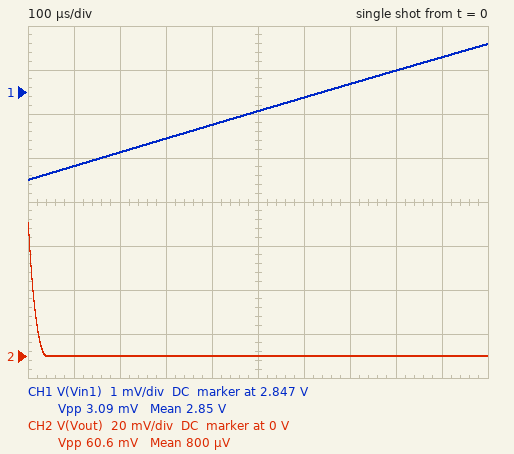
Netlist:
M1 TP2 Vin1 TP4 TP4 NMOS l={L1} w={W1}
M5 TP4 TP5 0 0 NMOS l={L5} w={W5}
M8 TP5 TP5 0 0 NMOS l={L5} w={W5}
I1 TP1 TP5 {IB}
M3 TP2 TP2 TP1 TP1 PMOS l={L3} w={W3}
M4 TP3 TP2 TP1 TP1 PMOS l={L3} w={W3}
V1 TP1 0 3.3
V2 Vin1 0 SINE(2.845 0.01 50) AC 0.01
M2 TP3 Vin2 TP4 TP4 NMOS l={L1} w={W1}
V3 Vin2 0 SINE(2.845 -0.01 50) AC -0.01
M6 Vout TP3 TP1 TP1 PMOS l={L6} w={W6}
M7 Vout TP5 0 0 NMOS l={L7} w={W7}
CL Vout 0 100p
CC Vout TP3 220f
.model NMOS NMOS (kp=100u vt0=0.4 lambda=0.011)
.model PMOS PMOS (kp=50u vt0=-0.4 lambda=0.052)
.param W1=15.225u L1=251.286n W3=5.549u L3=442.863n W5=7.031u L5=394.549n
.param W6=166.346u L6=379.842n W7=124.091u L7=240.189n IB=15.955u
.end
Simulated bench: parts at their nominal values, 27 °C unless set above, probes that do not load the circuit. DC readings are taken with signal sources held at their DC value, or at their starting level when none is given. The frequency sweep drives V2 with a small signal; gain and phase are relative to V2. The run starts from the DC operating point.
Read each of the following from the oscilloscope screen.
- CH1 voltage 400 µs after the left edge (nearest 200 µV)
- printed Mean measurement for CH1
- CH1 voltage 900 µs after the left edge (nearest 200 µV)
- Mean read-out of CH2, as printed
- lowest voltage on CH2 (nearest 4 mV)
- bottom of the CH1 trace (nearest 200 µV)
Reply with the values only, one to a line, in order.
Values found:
2.8462 V
2.85 V
2.8478 V
800 µV
0 V
2.8450 V
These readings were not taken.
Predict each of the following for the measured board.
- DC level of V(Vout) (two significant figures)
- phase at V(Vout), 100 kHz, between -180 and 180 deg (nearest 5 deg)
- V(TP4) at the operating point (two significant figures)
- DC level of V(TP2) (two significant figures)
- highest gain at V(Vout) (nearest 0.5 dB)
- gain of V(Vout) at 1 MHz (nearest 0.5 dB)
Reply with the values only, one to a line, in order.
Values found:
61 mV
150 deg
2.4 V
2.7 V
56.5 dB
41.0 dB
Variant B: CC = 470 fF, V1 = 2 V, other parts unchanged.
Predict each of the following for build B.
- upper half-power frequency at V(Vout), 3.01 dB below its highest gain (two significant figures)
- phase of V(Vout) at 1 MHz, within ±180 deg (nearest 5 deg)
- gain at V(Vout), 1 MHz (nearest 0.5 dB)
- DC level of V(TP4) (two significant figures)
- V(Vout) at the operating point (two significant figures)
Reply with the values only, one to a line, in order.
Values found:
5.8 MHz
170 deg
-58.0 dB
1.4 V
55 mV
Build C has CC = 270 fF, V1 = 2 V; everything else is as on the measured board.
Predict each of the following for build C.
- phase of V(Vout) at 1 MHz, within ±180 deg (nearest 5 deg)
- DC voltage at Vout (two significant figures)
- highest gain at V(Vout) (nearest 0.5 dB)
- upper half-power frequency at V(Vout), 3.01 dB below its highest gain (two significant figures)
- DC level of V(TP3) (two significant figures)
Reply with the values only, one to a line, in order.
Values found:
170 deg
55 mV
-58.0 dB
6.1 MHz
1.4 V
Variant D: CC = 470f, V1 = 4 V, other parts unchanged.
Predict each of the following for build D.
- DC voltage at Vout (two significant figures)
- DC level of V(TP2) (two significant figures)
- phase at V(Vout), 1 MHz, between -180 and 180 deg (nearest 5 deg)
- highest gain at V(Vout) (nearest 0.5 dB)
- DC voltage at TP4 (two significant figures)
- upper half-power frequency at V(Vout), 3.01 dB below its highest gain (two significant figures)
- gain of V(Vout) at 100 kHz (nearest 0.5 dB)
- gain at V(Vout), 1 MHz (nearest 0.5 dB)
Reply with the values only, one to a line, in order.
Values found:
63 mV
3.4 V
90 deg
57.5 dB
2.4 V
78 kHz
53.0 dB
35.0 dB
